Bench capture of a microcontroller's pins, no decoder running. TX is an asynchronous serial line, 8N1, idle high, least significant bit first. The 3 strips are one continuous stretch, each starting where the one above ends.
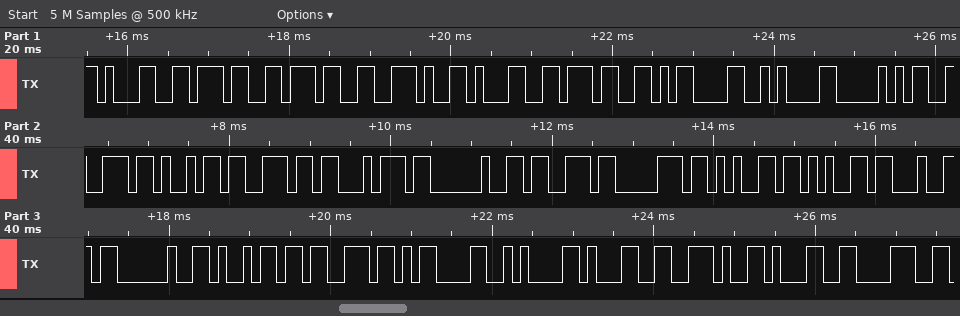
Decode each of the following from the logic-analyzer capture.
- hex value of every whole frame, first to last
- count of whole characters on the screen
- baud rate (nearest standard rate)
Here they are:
0x31 0x37 0x37 0x2E 0x31 0x37 0x0D 0x0A 0x50 0x72 0x69 0x6E 0x74 0x20 0x73 0x70 0x65 0x65 0x64 0x20 0x69 0x73 0x0D 0x0A 0x31 0x2E 0x31 0x38
28
9600 baud
